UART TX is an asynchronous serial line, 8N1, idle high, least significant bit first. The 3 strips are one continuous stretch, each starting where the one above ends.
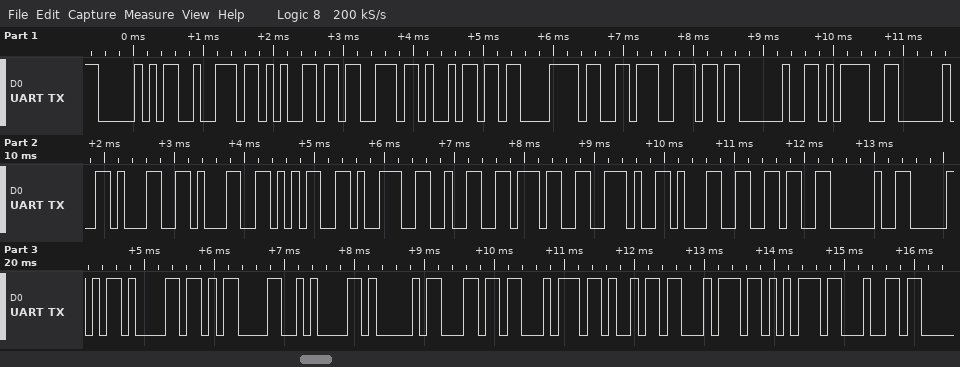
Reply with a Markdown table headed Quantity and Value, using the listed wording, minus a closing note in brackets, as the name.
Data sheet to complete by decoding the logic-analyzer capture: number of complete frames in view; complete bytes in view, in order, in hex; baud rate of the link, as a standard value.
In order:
| Quantity | Value |
|---|---|
| number of complete frames in view | 32 |
| complete bytes in view, in order, in hex | 50 72 65 73 69 C3 B3 6E 20 3D 20 31 31 35 39 32 37 2E 31 36 20 50 61 0D 0A 41 6C 74 69 74 75 64 |
| baud rate of the link, as a standard value | 9600 baud |
